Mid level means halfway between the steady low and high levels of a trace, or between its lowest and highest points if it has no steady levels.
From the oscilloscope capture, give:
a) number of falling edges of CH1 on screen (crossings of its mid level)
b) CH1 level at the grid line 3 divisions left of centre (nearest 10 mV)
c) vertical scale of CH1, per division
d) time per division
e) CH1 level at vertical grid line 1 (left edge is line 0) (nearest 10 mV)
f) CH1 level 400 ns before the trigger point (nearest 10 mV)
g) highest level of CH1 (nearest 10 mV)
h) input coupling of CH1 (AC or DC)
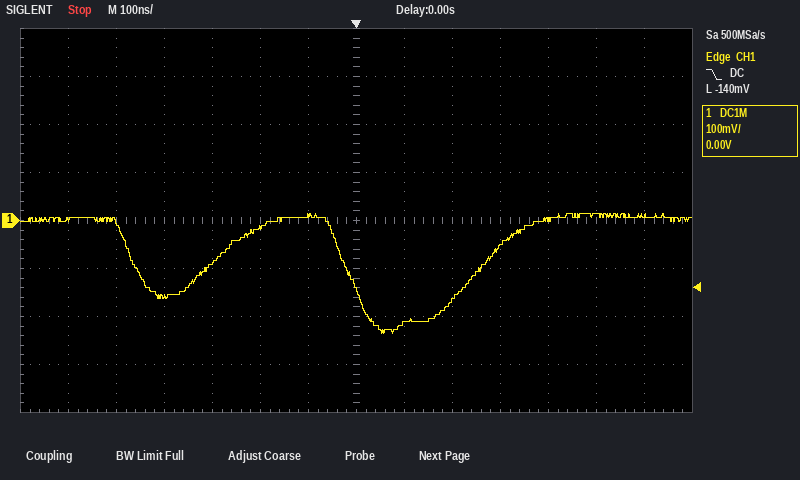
2
-90 mV
100 mV
100 ns
0 mV
-160 mV
10 mV
DC
